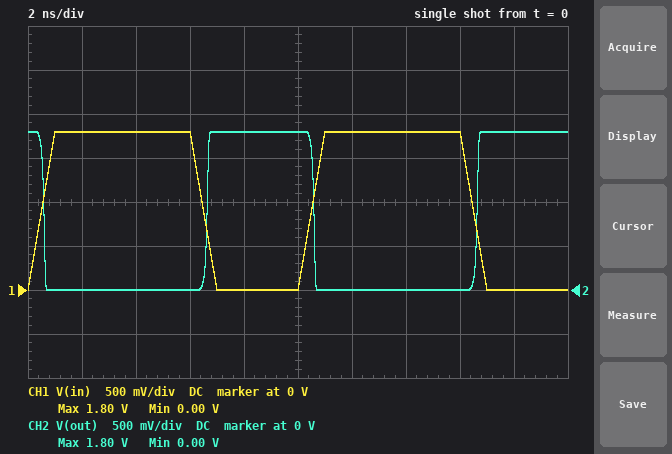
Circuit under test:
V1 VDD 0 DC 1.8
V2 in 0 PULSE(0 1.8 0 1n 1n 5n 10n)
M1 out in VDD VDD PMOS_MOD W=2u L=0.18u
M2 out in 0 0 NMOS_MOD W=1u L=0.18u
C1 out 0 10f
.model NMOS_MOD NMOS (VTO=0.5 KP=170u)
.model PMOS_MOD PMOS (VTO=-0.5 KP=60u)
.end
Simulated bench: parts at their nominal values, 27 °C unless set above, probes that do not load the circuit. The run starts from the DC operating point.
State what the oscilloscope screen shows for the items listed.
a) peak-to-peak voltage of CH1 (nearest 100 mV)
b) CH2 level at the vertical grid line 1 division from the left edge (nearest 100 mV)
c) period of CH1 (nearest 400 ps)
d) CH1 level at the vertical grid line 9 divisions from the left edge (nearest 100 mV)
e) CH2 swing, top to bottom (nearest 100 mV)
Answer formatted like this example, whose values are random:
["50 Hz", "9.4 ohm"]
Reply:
["1.8 V", "0 V", "10.0 ns", "0 V", "1.8 V"]
